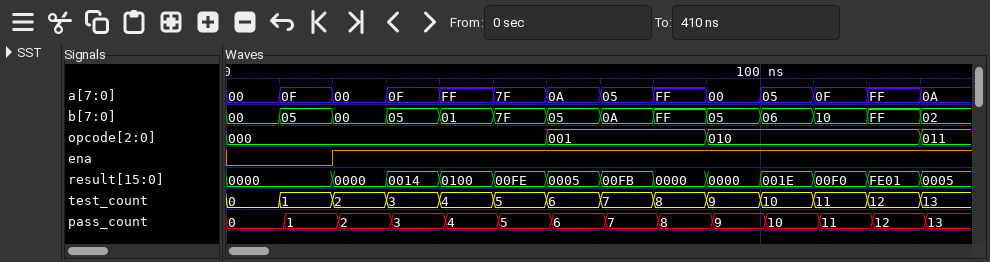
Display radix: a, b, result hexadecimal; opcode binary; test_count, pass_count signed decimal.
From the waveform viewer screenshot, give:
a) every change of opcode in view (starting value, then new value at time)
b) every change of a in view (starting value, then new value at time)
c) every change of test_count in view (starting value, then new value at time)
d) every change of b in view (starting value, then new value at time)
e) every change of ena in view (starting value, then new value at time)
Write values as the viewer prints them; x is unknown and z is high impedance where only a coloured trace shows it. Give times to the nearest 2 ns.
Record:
000, 001 at 60 ns, 010 at 90 ns, 011 at 130 ns
00, 0F at 10 ns, 00 at 20 ns, 0F at 30 ns, FF at 40 ns, 7F at 50 ns, 0A at 60 ns, 05 at 70 ns, FF at 80 ns, 00 at 90 ns, 05 at 100 ns, 0F at 110 ns, FF at 120 ns, 0A at 130 ns
0, 1 at 10 ns, 2 at 20 ns, 3 at 30 ns, 4 at 40 ns, 5 at 50 ns, 6 at 60 ns, 7 at 70 ns, 8 at 80 ns, 9 at 90 ns, 10 at 100 ns, 11 at 110 ns, 12 at 120 ns, 13 at 130 ns
00, 05 at 10 ns, 00 at 20 ns, 05 at 30 ns, 01 at 40 ns, 7F at 50 ns, 05 at 60 ns, 0A at 70 ns, FF at 80 ns, 05 at 90 ns, 06 at 100 ns, 10 at 110 ns, FF at 120 ns, 02 at 130 ns
0, 1 at 20 ns
